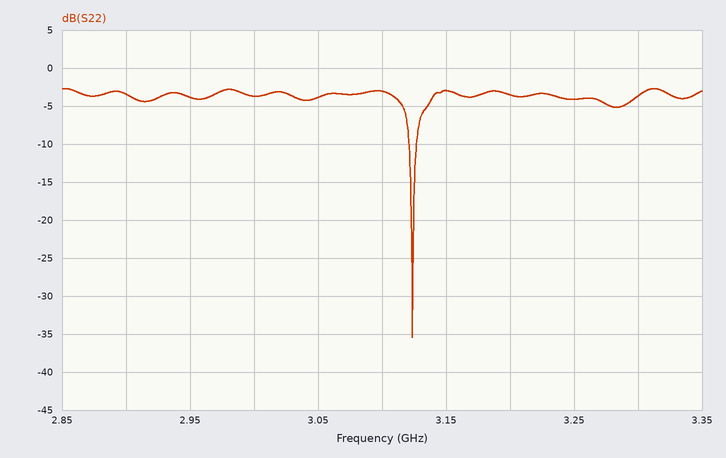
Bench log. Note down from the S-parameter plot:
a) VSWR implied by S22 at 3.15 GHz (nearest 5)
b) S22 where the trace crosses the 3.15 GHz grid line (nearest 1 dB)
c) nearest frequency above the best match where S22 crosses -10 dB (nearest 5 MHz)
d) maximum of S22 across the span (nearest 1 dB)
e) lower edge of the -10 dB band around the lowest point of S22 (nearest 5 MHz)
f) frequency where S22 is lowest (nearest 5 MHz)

5
-3 dB
3.125 GHz
-3 dB
3.120 GHz
3.125 GHz
